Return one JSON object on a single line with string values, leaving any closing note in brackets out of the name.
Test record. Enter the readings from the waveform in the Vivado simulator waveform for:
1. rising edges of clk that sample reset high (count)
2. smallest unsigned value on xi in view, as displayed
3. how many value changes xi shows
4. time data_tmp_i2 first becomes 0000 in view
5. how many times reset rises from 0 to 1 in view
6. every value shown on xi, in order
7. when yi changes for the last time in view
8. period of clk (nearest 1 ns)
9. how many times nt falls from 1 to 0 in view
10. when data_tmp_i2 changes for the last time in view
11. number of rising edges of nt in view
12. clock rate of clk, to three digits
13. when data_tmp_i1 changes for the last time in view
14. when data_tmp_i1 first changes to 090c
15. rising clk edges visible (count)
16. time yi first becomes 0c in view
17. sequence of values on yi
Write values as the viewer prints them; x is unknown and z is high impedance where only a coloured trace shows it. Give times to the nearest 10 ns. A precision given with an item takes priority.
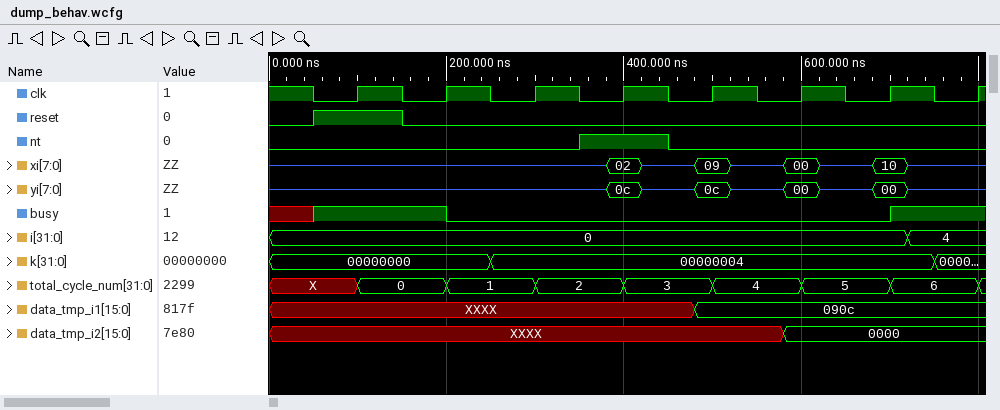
{"rising edges of clk that sample reset high": "1", "smallest unsigned value on xi in view, as displayed": "00", "how many value changes xi shows": "8", "time data_tmp_i2 first becomes 0000 in view": "580 ns", "how many times reset rises from 0 to 1 in view": "1", "every value shown on xi, in order": "z, 02, z, 09, z, 00, z, 10, z", "when yi changes for the last time in view": "720 ns", "period of clk": "100 ns", "how many times nt falls from 1 to 0 in view": "1", "when data_tmp_i2 changes for the last time in view": "580 ns", "number of rising edges of nt in view": "1", "clock rate of clk, to three digits": "10.0 MHz", "when data_tmp_i1 changes for the last time in view": "480 ns", "when data_tmp_i1 first changes to 090c": "480 ns", "rising clk edges visible": "8", "time yi first becomes 0c in view": "380 ns", "sequence of values on yi": "z, 0c, z, 0c, z, 00, z, 00, z"}
